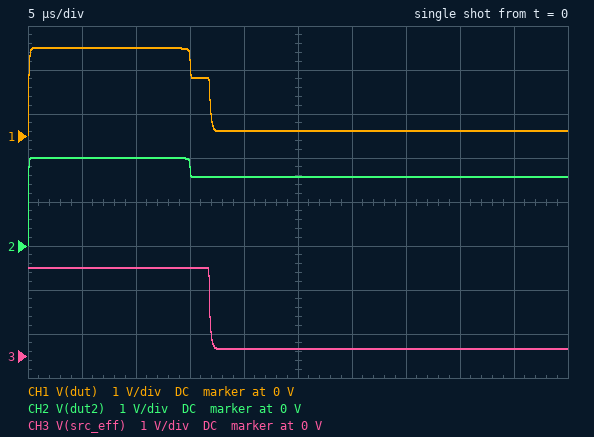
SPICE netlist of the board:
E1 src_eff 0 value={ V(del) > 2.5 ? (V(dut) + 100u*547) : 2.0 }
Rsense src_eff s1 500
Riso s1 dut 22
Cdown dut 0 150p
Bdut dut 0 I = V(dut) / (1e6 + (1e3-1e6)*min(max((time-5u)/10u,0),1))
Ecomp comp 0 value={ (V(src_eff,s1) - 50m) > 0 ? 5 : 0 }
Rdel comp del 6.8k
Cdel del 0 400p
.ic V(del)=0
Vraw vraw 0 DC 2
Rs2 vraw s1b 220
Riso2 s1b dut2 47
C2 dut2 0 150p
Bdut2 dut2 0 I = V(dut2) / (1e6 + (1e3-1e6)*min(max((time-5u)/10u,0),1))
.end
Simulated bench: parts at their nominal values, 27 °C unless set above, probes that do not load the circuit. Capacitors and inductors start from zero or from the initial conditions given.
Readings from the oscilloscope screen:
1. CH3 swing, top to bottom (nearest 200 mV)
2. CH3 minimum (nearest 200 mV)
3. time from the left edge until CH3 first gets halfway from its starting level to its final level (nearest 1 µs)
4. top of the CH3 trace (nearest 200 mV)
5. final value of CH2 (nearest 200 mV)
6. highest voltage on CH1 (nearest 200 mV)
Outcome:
1.8 V
200 mV
17 µs
2.0 V
1.6 V
2.0 V
